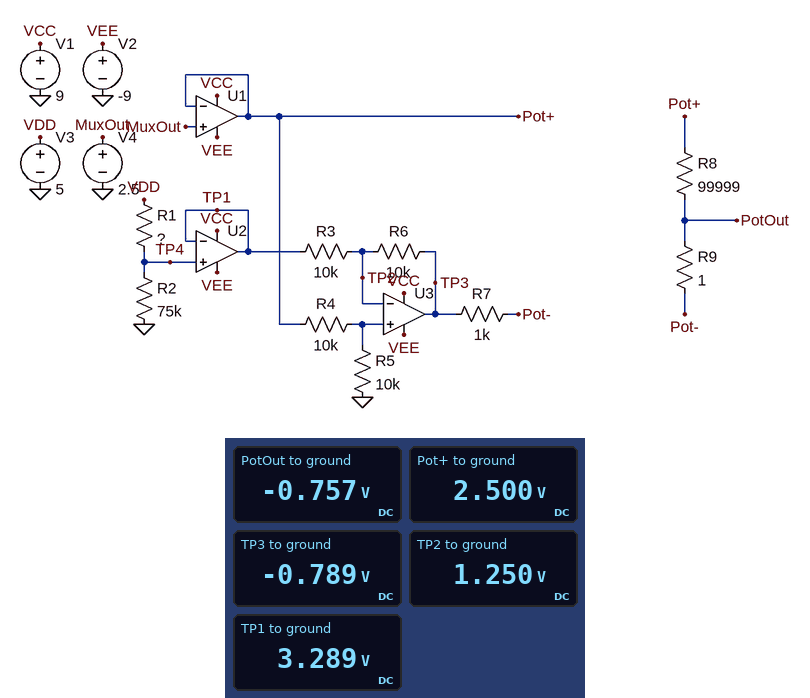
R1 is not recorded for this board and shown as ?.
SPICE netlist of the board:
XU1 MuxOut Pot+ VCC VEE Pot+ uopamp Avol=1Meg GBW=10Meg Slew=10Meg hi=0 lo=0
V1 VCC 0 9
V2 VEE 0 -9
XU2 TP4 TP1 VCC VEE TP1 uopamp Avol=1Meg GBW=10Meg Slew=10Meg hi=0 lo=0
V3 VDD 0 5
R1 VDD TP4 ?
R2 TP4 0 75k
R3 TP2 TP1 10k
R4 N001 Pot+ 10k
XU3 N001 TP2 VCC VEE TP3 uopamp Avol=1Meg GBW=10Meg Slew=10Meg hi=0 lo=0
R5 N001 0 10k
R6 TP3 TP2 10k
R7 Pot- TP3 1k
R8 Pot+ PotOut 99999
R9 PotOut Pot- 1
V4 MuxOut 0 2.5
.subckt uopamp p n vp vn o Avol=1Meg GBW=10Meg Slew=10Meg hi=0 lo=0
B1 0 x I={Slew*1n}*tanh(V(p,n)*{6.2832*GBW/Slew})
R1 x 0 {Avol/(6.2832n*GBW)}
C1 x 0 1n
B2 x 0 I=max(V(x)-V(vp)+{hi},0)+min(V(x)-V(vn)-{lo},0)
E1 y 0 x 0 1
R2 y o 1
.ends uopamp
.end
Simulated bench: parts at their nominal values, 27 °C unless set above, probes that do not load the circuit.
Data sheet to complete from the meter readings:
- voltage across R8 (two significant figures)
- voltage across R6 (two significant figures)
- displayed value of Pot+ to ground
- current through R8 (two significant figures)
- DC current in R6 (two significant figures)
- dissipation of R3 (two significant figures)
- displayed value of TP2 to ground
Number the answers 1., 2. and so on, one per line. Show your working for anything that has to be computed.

1. 2.5 V - (-757 mV) = 3.3 V
2. 1.25 V - (-789 mV) = 2.0 V
3. 2.500 V
4. (2.5 V - (-757 mV)) / 100 kΩ = 33 µA
5. (1.25 V - (-789 mV)) / 10 kΩ = 200 µA
6. (3.289 V - 1.25 V)^2 / 10 kΩ = 420 µW
7. 1.250 V
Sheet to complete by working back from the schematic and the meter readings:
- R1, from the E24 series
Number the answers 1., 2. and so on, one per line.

1. 39 kΩ
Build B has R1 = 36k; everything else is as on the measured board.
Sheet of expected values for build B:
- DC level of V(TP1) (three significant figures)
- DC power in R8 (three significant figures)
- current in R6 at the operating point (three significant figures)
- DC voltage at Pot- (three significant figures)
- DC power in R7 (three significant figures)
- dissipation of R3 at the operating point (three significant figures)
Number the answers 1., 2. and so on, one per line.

1. 3.38 V
2. 112 µW
3. 213 µA
4. -845 mV
5. 1.12 µW
6. 453 µW
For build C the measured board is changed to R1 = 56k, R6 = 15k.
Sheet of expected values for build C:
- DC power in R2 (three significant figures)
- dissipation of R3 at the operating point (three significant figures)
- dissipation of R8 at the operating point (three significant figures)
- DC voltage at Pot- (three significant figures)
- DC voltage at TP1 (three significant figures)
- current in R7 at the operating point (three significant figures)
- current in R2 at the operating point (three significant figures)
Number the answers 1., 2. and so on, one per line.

1. 109 µW
2. 260 µW
3. 132 µW
4. -1.13 V
5. 2.86 V
6. 36.3 µA
7. 38.2 µA
